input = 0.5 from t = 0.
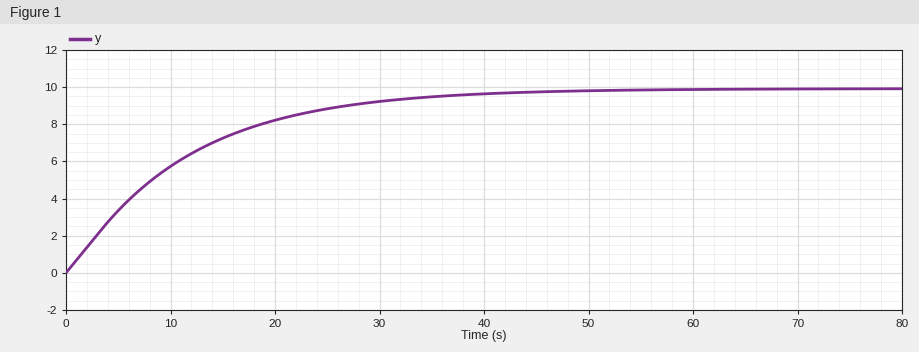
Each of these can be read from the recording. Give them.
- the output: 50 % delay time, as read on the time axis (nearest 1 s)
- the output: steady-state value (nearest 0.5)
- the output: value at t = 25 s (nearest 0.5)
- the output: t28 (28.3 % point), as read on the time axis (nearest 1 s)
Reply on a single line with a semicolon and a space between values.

8 s; 10.0; 9.0; 4 s
